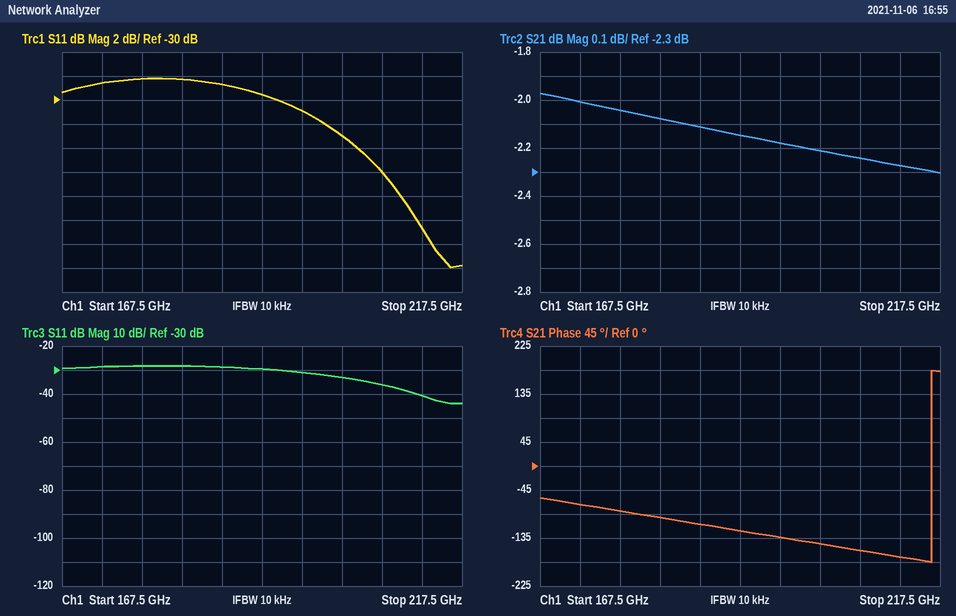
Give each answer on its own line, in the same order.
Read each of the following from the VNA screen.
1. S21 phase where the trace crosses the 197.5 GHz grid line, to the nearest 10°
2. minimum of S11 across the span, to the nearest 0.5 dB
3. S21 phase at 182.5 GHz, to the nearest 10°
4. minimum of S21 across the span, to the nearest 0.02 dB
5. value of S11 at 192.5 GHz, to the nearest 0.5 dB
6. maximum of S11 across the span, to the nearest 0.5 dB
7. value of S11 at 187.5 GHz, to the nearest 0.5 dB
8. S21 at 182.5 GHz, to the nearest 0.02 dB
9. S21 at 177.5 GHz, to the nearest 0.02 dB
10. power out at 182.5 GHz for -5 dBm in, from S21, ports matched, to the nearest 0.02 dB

-130°
-44.0 dB
-100°
-2.30 dB
-29.5 dB
-28.0 dB
-28.5 dB
-2.08 dB
-2.04 dB
-7.08 dBm
